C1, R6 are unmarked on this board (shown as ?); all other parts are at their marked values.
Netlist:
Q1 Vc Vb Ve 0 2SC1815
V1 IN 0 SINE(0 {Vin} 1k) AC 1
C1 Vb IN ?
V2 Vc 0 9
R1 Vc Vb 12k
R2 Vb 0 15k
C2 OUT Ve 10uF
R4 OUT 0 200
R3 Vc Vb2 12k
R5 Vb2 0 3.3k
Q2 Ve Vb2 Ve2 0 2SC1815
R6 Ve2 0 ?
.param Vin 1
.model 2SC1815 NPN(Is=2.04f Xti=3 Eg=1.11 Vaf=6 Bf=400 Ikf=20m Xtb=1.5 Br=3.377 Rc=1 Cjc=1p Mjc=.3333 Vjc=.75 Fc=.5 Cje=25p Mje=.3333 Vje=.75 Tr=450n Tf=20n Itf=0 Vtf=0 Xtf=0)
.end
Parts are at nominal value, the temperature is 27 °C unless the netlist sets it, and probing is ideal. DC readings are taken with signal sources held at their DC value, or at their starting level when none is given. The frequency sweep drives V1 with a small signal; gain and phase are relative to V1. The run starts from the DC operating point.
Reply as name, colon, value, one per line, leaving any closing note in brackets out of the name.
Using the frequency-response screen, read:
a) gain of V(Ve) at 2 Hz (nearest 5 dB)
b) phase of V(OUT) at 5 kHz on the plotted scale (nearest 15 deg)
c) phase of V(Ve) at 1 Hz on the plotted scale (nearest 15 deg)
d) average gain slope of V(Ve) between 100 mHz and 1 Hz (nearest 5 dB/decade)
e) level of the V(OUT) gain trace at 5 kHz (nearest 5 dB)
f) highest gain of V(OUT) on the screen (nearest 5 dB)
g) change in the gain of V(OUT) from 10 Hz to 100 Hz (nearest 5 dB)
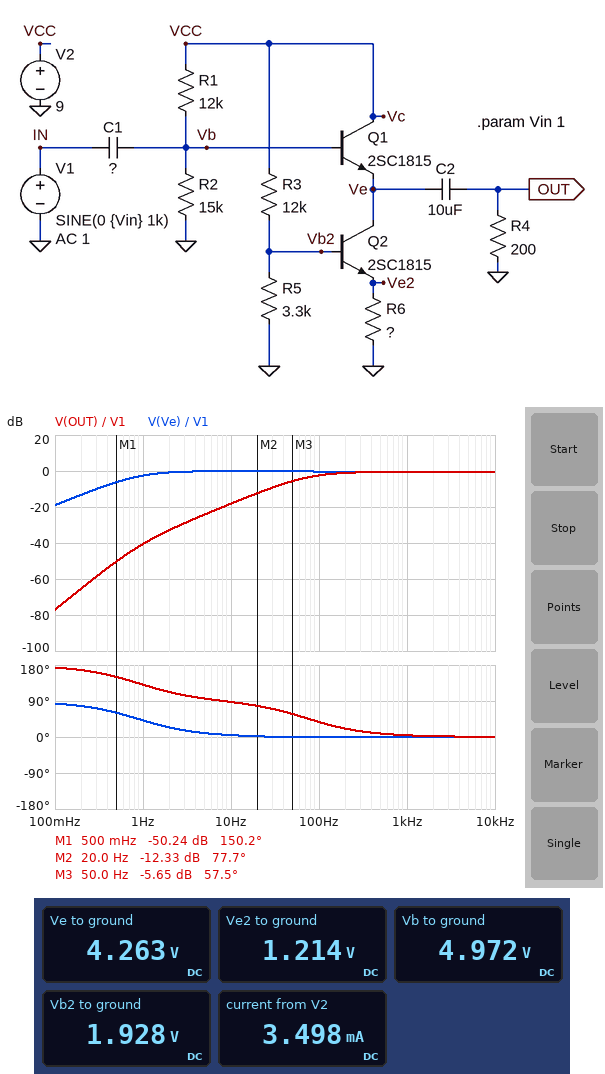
gain of V(Ve) at 2 Hz: 0 dB
phase of V(OUT) at 5 kHz on the plotted scale: 0 deg
phase of V(Ve) at 1 Hz on the plotted scale: 45 deg
average gain slope of V(Ve) between 100 mHz and 1 Hz: 15 dB/decade
level of the V(OUT) gain trace at 5 kHz: 0 dB
highest gain of V(OUT) on the screen: 0 dB
change in the gain of V(OUT) from 10 Hz to 100 Hz: 15 dB
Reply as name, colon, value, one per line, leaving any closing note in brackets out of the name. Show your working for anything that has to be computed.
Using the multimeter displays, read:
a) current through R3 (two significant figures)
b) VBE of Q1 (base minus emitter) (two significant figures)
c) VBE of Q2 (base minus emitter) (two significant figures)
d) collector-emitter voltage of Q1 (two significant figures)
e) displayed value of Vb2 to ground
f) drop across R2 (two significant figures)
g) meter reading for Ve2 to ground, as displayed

current through R3: (9 V - 1.928 V) / 12 kΩ = 590 µA
VBE of Q1 (base minus emitter): 4.972 V - 4.263 V = 710 mV
VBE of Q2 (base minus emitter): 1.928 V - 1.214 V = 710 mV
collector-emitter voltage of Q1: 9 V - 4.263 V = 4.7 V
displayed value of Vb2 to ground: 1.928 V
drop across R2: 4.972 V = 5.0 V
meter reading for Ve2 to ground, as displayed: 1.214 V
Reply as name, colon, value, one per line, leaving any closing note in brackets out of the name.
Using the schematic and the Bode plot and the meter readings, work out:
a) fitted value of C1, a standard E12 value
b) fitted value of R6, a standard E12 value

fitted value of C1, a standard E12 value: 27 µF
fitted value of R6, a standard E12 value: 470 Ω
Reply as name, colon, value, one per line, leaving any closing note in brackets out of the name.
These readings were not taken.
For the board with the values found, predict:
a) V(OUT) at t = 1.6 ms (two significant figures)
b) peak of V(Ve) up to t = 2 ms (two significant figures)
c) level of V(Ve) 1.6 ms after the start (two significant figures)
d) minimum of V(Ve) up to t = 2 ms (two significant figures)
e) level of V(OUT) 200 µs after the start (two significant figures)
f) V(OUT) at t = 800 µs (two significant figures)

V(OUT) at t = 1.6 ms: -510 mV
peak of V(Ve) up to t = 2 ms: 5.2 V
level of V(Ve) 1.6 ms after the start: 3.9 V
minimum of V(Ve) up to t = 2 ms: 3.8 V
level of V(OUT) 200 µs after the start: 870 mV
V(OUT) at t = 800 µs: -510 mV
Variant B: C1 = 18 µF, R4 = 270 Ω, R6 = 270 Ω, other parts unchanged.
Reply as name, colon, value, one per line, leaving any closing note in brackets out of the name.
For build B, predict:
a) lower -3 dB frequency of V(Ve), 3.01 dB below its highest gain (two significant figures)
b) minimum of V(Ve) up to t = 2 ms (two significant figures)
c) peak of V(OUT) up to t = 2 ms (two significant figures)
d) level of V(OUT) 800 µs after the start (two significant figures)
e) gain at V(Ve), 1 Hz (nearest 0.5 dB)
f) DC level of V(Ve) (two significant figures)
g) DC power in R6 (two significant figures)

lower -3 dB frequency of V(Ve), 3.01 dB below its highest gain: 1.3 Hz
minimum of V(Ve) up to t = 2 ms: 3.3 V
peak of V(OUT) up to t = 2 ms: 940 mV
level of V(OUT) 800 µs after the start: -930 mV
gain at V(Ve), 1 Hz: -4.5 dB
DC level of V(Ve): 4.2 V
DC power in R6: 5.2 mW
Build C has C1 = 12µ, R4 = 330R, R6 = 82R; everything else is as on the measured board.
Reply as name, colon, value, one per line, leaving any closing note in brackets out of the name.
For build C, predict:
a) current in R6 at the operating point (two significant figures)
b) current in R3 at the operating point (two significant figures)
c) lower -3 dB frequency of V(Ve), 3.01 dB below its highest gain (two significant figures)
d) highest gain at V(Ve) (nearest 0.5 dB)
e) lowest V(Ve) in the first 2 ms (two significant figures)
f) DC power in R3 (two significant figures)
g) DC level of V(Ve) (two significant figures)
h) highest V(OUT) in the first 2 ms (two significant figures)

current in R6 at the operating point: 13 mA
current in R3 at the operating point: 600 µA
lower -3 dB frequency of V(Ve), 3.01 dB below its highest gain: 2.0 Hz
highest gain at V(Ve): 0 dB
lowest V(Ve) in the first 2 ms: 3.1 V
DC power in R3: 4.3 mW
DC level of V(Ve): 4.1 V
highest V(OUT) in the first 2 ms: 950 mV
